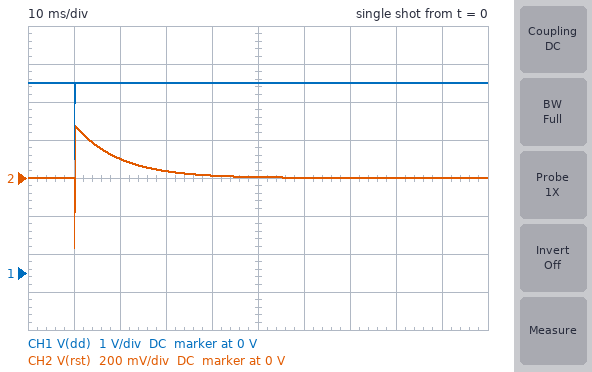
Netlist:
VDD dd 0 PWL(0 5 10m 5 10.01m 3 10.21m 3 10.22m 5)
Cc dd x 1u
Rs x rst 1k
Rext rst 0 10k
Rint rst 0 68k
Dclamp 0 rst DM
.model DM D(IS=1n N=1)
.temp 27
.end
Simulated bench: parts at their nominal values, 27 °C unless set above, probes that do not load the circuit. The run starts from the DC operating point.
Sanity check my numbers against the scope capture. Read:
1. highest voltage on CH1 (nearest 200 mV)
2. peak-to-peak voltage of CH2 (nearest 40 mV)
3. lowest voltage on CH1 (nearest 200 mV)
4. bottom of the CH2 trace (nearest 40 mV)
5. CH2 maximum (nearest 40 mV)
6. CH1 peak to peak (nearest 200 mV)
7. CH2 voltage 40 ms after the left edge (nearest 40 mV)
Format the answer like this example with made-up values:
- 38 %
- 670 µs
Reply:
- 5.0 V
- 640 mV
- 3.0 V
- -360 mV
- 280 mV
- 2.0 V
- 0 V
